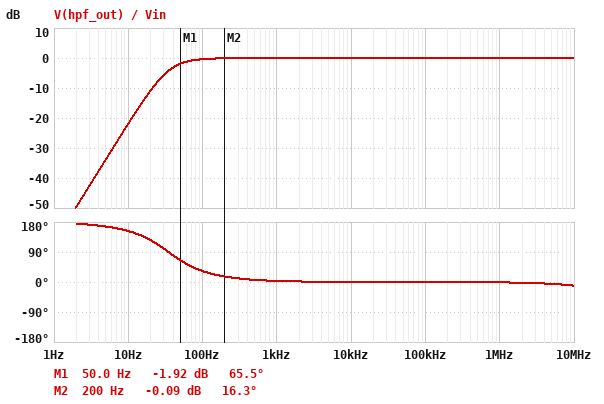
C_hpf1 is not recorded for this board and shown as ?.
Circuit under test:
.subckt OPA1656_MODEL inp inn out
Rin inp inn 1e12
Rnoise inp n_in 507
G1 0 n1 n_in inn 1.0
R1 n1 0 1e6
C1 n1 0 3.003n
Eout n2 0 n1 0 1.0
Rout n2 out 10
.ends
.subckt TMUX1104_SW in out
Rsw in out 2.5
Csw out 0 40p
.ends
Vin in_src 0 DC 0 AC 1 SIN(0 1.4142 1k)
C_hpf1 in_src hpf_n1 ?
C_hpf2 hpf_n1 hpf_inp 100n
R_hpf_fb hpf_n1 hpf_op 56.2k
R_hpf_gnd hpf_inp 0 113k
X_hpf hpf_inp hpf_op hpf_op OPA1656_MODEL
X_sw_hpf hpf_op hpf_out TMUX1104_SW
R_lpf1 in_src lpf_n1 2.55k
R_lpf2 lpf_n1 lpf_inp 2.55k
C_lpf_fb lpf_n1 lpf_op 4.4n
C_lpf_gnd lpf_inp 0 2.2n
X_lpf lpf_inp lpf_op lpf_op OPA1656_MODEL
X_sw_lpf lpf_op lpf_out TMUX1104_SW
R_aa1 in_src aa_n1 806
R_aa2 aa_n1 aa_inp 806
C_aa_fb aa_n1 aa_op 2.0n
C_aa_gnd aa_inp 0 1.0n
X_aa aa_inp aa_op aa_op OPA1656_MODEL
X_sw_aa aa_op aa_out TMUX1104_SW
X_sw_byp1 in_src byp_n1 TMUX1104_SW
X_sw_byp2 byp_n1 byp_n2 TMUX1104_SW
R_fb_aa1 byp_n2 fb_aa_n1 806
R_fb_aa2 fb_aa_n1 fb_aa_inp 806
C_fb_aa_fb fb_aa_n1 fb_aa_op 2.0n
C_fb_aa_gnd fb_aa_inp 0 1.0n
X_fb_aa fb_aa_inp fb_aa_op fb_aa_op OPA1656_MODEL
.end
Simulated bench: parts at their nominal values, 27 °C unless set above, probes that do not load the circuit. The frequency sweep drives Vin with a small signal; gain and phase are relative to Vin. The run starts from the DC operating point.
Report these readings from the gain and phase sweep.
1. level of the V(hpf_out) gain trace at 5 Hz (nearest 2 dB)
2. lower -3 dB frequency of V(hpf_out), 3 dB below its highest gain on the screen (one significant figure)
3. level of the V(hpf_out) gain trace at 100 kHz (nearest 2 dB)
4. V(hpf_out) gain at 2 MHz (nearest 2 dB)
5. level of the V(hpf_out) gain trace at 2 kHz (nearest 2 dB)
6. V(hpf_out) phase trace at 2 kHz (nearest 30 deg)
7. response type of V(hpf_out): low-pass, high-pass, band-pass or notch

-34 dB
40 Hz
0 dB
0 dB
0 dB
0 deg
high-pass
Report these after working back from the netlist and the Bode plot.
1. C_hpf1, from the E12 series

33 nF
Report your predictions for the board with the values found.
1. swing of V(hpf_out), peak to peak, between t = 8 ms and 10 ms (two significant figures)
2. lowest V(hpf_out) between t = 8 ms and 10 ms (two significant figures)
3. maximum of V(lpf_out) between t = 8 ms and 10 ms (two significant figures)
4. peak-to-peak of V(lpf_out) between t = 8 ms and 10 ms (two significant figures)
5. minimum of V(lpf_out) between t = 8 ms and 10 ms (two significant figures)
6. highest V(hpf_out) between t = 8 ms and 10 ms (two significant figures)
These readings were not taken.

2.8 V
-1.4 V
1.4 V
2.8 V
-1.4 V
1.4 V
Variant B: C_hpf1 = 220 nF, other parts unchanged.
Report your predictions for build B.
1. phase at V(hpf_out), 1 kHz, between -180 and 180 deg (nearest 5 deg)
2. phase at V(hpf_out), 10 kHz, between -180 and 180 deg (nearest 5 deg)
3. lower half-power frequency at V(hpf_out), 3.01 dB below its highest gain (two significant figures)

0 deg
0 deg
15 Hz
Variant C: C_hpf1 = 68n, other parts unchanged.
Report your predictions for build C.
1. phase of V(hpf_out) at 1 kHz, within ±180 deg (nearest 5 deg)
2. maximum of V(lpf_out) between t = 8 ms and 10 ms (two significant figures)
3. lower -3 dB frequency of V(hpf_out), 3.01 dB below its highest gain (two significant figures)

0 deg
1.4 V
25 Hz
